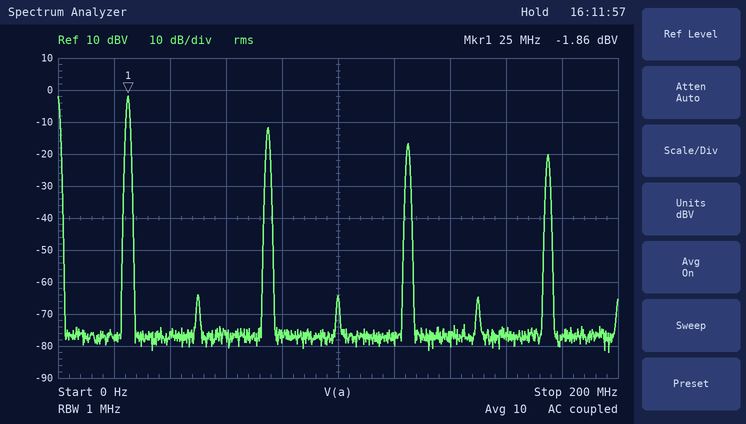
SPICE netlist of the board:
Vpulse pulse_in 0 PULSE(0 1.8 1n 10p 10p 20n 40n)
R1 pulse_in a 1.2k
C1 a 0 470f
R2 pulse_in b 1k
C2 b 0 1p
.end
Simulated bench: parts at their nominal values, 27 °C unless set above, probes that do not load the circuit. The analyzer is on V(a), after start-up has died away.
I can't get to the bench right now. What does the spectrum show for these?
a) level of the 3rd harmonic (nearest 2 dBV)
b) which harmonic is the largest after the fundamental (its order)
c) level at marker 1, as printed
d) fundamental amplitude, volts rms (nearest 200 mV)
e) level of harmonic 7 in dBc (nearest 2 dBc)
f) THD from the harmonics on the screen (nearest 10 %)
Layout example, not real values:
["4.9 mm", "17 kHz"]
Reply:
["-12 dBV", "3", "-1.86 dBV", "800 mV", "-18 dBc", "40 %"]
